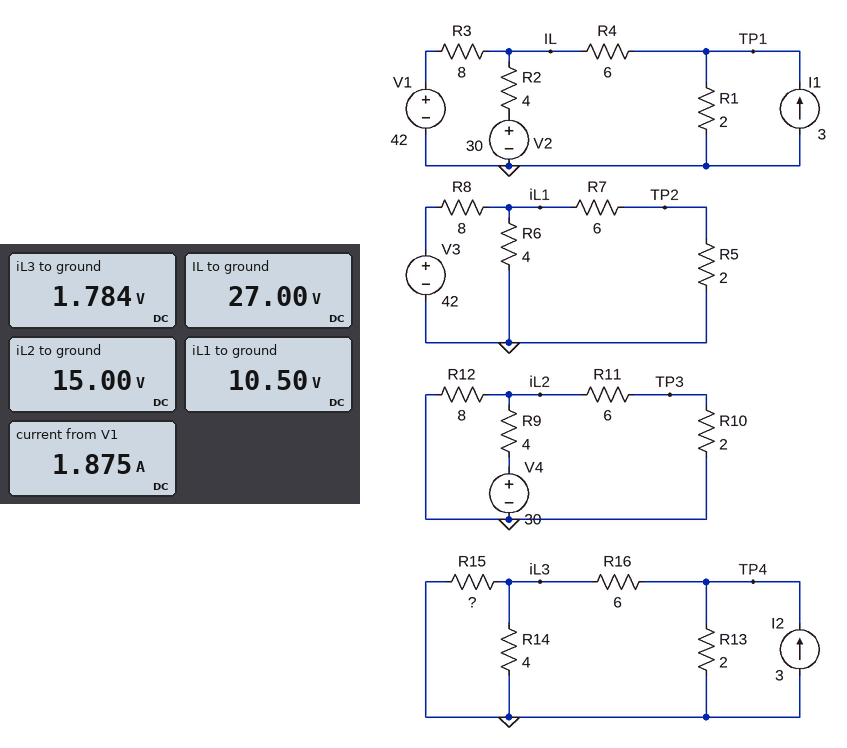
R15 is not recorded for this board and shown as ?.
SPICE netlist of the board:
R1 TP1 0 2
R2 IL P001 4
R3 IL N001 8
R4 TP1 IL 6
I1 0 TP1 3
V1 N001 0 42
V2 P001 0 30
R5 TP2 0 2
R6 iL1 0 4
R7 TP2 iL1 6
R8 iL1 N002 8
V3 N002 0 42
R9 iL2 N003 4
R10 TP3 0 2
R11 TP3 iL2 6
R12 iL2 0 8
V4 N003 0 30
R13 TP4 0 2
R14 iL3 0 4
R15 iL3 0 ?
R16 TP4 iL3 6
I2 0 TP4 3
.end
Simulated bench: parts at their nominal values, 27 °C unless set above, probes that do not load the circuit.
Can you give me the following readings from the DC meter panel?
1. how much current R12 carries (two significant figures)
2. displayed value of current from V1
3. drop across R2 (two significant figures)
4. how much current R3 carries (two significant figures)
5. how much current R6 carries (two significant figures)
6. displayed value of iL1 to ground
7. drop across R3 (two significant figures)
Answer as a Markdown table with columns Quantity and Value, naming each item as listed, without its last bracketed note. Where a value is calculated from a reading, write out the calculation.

| Quantity | Value |
|---|---|
| how much current R12 carries | (15 V) / 8 Ω = 1.9 A |
| displayed value of current from V1 | 1.875 A |
| drop across R2 | 30 V - 27 V = 3.0 V |
| how much current R3 carries | (42 V - 27 V) / 8 Ω = 1.9 A |
| how much current R6 carries | (10.5 V) / 4 Ω = 2.6 A |
| displayed value of iL1 to ground | 10.50 V |
| drop across R3 | 42 V - 27 V = 15 V |
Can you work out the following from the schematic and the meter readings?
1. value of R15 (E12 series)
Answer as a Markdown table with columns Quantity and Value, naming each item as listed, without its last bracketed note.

| Quantity | Value |
|---|---|
| value of R15 | 22 Ω |
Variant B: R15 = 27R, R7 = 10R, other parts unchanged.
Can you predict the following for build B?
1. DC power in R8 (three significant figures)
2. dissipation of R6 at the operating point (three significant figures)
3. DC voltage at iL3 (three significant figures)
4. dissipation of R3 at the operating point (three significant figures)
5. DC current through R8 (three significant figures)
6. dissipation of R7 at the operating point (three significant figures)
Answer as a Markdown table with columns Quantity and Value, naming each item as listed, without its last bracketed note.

| Quantity | Value |
|---|---|
| DC power in R8 | 117 W |
| dissipation of R6 at the operating point | 32.8 W |
| DC voltage at iL3 | 1.82 V |
| dissipation of R3 at the operating point | 28.1 W |
| DC current through R8 | 3.82 A |
| dissipation of R7 at the operating point | 9.11 W |
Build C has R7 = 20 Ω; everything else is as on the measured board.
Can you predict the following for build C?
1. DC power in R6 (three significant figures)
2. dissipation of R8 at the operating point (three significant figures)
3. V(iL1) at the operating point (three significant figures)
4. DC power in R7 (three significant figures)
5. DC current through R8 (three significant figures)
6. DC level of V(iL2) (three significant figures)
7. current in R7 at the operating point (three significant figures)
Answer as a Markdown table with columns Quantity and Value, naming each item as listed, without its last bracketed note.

| Quantity | Value |
|---|---|
| DC power in R6 | 39.0 W |
| dissipation of R8 at the operating point | 109 W |
| V(iL1) at the operating point | 12.5 V |
| DC power in R7 | 6.44 W |
| DC current through R8 | 3.69 A |
| DC level of V(iL2) | 15.0 V |
| current in R7 at the operating point | 568 mA |
